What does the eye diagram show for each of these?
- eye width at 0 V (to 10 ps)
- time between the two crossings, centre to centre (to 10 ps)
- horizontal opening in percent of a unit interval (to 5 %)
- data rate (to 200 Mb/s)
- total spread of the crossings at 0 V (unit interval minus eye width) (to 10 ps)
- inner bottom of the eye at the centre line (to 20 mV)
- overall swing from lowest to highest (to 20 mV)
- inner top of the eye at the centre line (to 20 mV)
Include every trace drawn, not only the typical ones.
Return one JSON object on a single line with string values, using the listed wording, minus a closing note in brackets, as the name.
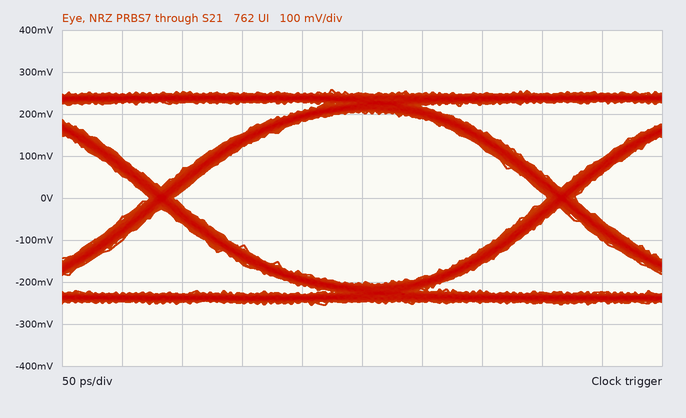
{"eye width at 0 V": "310 ps", "time between the two crossings, centre to centre": "330 ps", "horizontal opening in percent of a unit interval": "95 %", "data rate": "3.0 Gb/s", "total spread of the crossings at 0 V (unit interval minus eye width)": "20 ps", "inner bottom of the eye at the centre line": "-200 mV", "overall swing from lowest to highest": "520 mV", "inner top of the eye at the centre line": "200 mV"}
